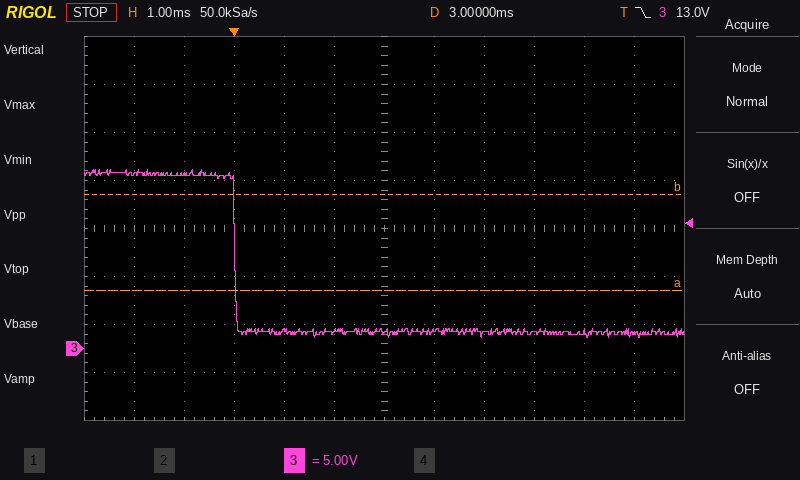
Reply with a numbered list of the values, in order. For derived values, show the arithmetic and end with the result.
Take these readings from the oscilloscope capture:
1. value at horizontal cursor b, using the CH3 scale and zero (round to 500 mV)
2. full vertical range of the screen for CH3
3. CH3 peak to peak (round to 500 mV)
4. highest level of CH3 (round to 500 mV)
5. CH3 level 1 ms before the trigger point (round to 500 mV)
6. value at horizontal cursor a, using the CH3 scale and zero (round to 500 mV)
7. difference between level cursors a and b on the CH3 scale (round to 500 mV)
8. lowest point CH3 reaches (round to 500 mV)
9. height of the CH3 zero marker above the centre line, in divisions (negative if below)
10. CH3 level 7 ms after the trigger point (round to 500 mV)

1. 16.0 V
2. 40 V
3. 18.5 V − (1.0 V) = 17.5 V
4. 18.5 V
5. 18.0 V
6. 6.0 V
7. 10.0 V
8. 1.0 V
9. -2.5 div
10. 1.5 V
